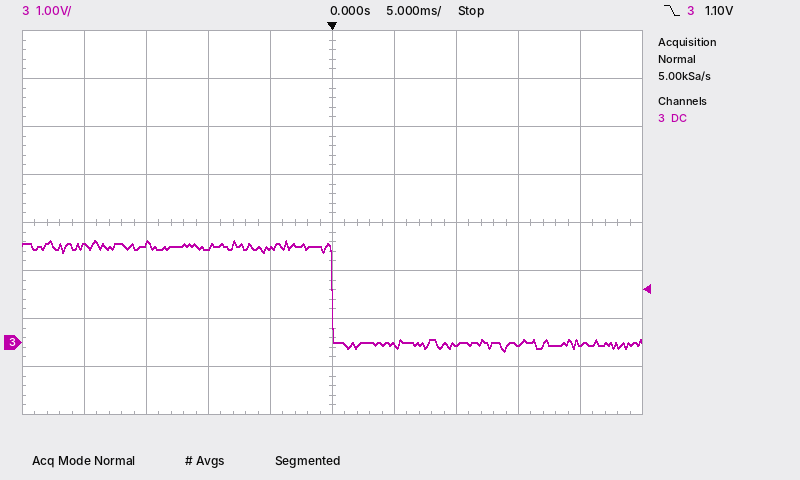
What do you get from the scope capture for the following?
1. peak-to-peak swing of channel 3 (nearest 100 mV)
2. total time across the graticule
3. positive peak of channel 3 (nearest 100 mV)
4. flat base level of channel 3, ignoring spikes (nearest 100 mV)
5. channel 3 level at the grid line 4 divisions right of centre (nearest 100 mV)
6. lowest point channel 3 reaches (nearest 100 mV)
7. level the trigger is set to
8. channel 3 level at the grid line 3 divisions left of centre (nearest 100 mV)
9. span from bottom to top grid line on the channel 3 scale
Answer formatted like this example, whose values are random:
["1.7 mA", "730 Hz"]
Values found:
["2.3 V", "50 ms", "2.1 V", "0.0 V", "0.0 V", "-200 mV", "1.10 V", "2.1 V", "8 V"]
